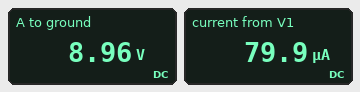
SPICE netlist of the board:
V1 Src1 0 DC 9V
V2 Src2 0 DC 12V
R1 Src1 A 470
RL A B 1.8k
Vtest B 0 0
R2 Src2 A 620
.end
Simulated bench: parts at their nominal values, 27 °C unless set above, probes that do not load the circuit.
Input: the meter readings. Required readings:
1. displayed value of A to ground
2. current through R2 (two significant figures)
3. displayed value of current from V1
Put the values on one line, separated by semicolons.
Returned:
8.96 V; 4.9 mA; 79.9 µA
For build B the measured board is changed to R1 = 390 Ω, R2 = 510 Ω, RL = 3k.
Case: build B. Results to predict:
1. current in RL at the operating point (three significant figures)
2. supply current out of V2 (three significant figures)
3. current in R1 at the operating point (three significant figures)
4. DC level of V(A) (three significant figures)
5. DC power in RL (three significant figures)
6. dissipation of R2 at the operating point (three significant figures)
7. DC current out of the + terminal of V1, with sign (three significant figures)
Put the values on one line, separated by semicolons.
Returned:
3.20 mA; 4.72 mA; 1.52 mA; 9.59 V; 30.7 mW; 11.4 mW; -1.52 mA
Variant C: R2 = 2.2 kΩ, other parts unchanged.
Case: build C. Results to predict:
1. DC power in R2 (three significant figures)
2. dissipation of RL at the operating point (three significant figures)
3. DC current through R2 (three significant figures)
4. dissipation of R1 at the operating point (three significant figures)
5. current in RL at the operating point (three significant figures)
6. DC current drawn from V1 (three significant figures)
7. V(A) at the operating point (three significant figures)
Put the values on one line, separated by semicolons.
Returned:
7.86 mW; 34.2 mW; 1.89 mA; 2.86 mW; 4.36 mA; 2.47 mA; 7.84 V
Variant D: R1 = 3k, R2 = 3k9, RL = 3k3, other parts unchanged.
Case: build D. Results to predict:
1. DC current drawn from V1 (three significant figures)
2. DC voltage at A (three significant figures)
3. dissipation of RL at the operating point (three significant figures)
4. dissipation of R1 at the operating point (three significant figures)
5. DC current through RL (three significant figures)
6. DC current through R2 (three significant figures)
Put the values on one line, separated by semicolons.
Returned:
731 µA; 6.81 V; 14.0 mW; 1.60 mW; 2.06 mA; 1.33 mA
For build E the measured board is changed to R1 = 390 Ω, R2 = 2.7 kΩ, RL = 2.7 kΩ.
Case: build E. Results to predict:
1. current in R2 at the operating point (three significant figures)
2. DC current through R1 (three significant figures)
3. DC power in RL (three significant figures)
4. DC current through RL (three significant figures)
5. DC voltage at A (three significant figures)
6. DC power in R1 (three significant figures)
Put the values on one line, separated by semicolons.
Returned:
1.36 mA; 1.72 mA; 25.7 mW; 3.08 mA; 8.33 V; 1.16 mW
